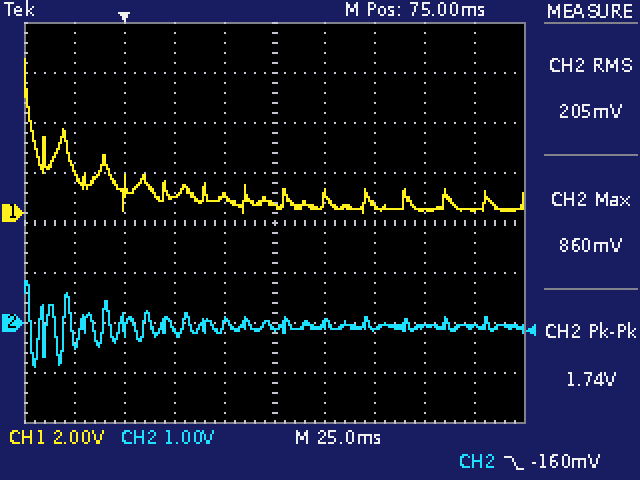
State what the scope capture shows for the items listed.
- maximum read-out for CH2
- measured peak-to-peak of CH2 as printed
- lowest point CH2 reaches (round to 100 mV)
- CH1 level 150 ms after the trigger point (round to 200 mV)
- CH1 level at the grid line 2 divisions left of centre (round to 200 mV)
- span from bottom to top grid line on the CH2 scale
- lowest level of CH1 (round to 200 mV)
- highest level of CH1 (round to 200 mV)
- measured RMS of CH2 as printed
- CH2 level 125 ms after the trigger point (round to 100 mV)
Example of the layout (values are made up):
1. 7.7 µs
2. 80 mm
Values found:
1. 860 mV
2. 1.74 V
3. -900 mV
4. 200 mV
5. 600 mV
6. 8 V
7. 0.0 V
8. 6.2 V
9. 205 mV
10. -100 mV
